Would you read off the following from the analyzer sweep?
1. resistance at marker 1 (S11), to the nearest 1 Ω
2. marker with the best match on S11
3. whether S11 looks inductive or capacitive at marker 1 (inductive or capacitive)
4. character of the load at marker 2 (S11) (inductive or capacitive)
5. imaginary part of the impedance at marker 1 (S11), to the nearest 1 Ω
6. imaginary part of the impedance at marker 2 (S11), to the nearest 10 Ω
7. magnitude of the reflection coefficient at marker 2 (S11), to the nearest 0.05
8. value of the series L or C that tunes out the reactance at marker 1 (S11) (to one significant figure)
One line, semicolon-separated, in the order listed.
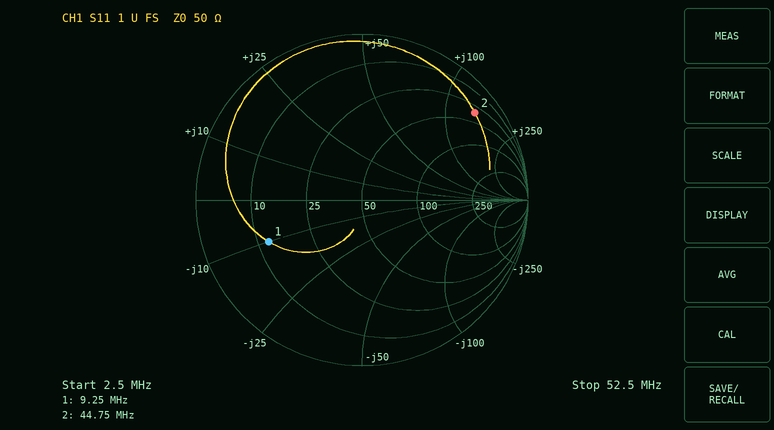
12 Ω; marker 1; capacitive; inductive; -10 Ω; +140 Ω; 0.85; 200 nH
